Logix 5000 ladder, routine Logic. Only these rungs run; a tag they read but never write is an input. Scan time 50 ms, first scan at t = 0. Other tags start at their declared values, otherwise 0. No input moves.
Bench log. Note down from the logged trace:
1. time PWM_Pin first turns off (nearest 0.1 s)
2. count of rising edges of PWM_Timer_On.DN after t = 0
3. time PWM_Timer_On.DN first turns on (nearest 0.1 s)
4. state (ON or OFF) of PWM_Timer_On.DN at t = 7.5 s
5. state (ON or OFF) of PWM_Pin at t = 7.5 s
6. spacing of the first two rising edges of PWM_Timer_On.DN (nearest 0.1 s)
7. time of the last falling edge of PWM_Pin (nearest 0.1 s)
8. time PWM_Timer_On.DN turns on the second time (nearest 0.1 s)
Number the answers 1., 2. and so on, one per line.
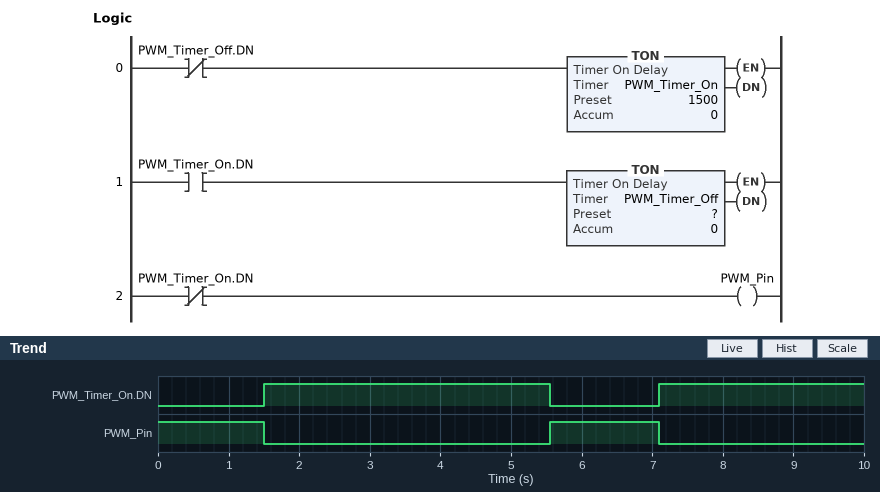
1. 1.5 s
2. 2
3. 1.5 s
4. ON
5. OFF
6. 5.6 s
7. 7.1 s
8. 7.1 s
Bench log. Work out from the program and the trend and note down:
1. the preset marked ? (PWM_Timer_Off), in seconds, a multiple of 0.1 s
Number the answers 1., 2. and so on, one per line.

1. 4.0 s
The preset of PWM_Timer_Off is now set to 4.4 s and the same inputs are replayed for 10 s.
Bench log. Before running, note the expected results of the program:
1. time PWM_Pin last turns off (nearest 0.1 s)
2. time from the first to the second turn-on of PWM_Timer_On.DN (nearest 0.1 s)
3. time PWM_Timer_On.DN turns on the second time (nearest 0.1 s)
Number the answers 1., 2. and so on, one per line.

1. 7.5 s
2. 6.0 s
3. 7.5 s
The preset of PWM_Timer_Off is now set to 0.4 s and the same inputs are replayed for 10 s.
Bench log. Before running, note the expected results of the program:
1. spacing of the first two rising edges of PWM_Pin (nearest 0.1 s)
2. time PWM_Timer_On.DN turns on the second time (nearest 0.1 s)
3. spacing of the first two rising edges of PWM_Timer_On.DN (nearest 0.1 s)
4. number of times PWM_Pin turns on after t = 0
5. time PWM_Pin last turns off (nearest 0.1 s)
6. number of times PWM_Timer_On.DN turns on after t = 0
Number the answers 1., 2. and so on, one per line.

1. 2.0 s
2. 3.5 s
3. 2.0 s
4. 5
5. 9.5 s
6. 5
